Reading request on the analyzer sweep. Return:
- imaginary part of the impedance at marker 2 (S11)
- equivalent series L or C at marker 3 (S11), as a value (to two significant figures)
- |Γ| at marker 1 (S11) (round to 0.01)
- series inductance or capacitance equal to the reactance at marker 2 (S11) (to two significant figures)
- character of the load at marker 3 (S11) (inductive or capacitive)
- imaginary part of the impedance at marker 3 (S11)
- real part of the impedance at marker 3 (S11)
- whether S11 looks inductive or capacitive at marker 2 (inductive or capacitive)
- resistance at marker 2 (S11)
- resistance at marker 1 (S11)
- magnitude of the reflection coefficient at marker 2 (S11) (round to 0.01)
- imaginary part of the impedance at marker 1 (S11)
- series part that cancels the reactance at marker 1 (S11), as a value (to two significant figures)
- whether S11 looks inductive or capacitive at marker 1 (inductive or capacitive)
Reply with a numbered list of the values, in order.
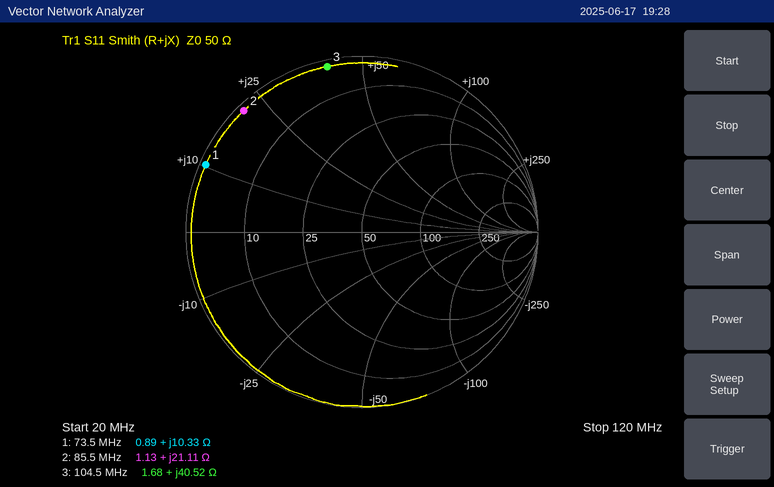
1. +21.11 Ω
2. 62 nH
3. 0.97
4. 39 nH
5. inductive
6. +40.52 Ω
7. 1.68 Ω
8. inductive
9. 1.13 Ω
10. 0.89 Ω
11. 0.96
12. +10.33 Ω
13. 210 pF
14. inductive
